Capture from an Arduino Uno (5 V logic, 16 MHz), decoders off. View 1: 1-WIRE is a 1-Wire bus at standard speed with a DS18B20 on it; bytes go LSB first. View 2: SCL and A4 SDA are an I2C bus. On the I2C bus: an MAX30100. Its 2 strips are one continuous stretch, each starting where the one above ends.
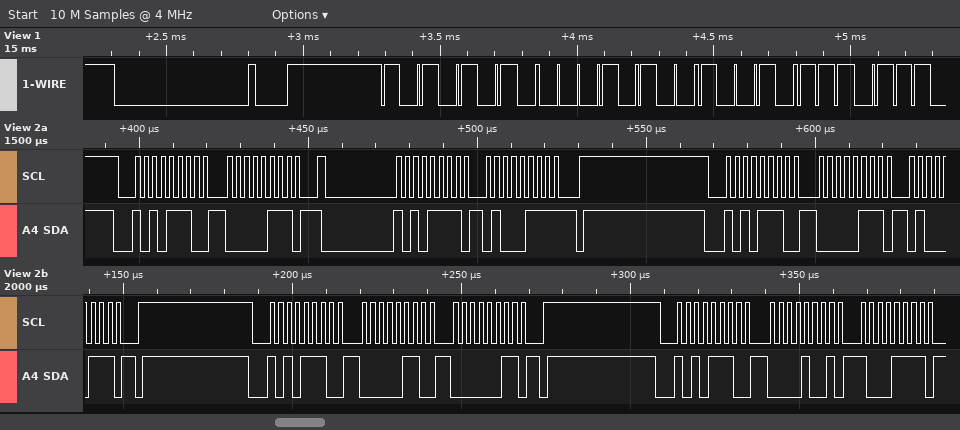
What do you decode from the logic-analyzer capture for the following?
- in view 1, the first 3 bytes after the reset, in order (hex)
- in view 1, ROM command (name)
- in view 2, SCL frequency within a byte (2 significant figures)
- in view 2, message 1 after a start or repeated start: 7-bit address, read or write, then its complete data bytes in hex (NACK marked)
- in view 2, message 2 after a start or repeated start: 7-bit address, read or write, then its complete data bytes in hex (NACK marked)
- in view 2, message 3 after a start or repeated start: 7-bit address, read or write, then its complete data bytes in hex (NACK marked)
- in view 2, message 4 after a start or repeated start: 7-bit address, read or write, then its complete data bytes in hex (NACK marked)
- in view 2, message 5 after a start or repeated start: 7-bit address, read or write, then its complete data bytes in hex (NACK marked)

55 28 E9
Match ROM
400 kHz
0x57 write: 07
0x57 read: 47 NACK
0x57 write: 07 47
0x57 write: 06 03
0x57 write: 09 8F
